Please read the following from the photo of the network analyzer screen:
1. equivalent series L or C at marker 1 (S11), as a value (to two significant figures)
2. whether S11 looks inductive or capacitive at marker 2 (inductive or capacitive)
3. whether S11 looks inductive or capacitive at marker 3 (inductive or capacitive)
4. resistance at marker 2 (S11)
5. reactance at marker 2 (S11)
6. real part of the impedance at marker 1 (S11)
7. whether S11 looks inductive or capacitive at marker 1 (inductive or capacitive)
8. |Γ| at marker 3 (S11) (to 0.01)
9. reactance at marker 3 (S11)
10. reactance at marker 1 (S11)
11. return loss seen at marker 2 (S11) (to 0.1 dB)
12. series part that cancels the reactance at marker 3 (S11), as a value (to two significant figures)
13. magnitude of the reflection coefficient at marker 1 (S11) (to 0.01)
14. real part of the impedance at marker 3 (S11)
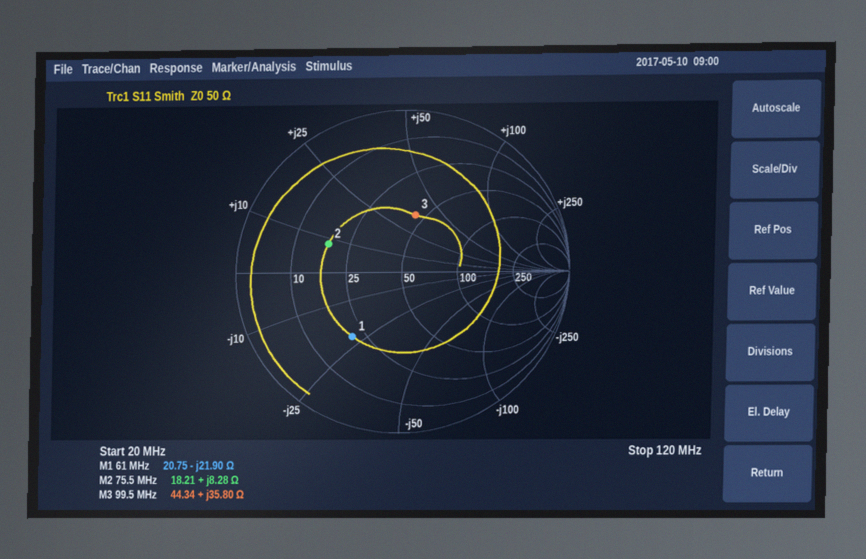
120 pF
inductive
inductive
18.21 Ω
+8.28 Ω
20.75 Ω
capacitive
0.36
+35.80 Ω
-21.90 Ω
6.4 dB
45 pF
0.49
44.34 Ω
